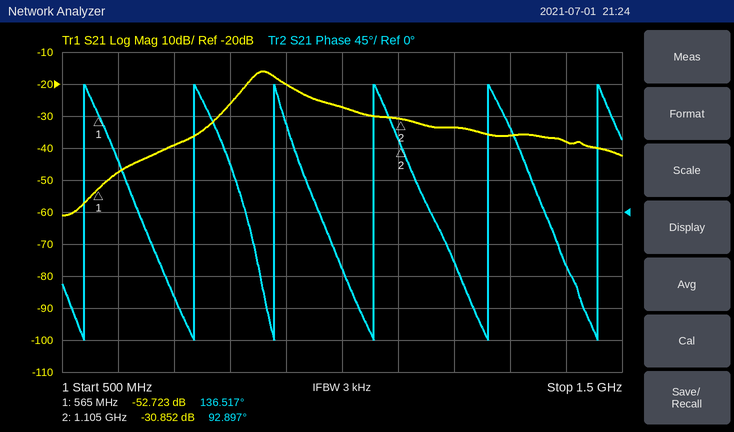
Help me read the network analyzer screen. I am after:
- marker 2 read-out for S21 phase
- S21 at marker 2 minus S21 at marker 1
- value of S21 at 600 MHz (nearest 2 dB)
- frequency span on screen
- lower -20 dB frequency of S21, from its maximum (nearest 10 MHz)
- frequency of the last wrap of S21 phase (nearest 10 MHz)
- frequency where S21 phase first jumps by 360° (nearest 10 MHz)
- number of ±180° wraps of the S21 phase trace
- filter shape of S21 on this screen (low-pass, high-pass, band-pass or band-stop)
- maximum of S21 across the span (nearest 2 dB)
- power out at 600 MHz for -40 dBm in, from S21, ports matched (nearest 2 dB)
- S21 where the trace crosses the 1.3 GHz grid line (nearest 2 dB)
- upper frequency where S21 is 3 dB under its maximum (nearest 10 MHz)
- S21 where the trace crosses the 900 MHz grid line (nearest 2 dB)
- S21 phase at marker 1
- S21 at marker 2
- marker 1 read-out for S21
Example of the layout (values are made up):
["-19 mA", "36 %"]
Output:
["92.897°", "21.871 dB", "-48 dB", "1 GHz", "740 MHz", "1.46 GHz", "540 MHz", "6", "band-pass", "-16 dB", "-88 dBm", "-36 dB", "890 MHz", "-20 dB", "136.517°", "-30.852 dB", "-52.723 dB"]
